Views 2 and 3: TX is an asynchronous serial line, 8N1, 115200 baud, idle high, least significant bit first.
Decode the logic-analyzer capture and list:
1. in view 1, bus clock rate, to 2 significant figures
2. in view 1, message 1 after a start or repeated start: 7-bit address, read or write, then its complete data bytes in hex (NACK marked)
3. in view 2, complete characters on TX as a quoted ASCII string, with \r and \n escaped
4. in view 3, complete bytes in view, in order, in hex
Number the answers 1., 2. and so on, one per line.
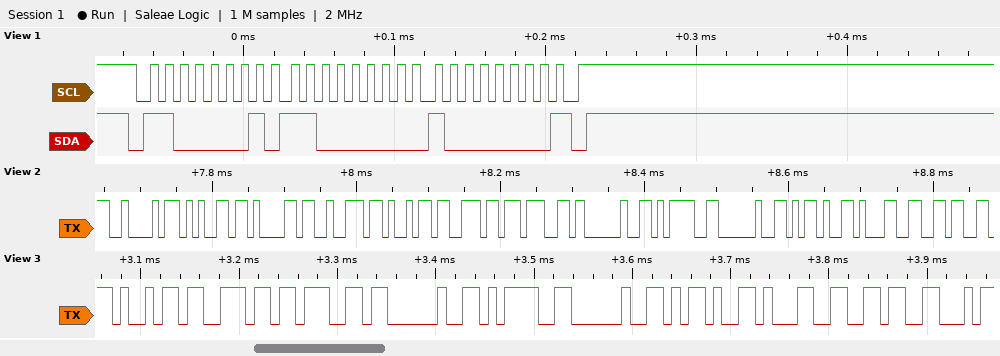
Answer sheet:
1. 100 kHz
2. 0x60 read: C0 80 NACK
3. "Bearing = -16"
4. 0x69 0x6E 0x67 0x20 0x3D 0x20 0x2D 0x31 0x36
